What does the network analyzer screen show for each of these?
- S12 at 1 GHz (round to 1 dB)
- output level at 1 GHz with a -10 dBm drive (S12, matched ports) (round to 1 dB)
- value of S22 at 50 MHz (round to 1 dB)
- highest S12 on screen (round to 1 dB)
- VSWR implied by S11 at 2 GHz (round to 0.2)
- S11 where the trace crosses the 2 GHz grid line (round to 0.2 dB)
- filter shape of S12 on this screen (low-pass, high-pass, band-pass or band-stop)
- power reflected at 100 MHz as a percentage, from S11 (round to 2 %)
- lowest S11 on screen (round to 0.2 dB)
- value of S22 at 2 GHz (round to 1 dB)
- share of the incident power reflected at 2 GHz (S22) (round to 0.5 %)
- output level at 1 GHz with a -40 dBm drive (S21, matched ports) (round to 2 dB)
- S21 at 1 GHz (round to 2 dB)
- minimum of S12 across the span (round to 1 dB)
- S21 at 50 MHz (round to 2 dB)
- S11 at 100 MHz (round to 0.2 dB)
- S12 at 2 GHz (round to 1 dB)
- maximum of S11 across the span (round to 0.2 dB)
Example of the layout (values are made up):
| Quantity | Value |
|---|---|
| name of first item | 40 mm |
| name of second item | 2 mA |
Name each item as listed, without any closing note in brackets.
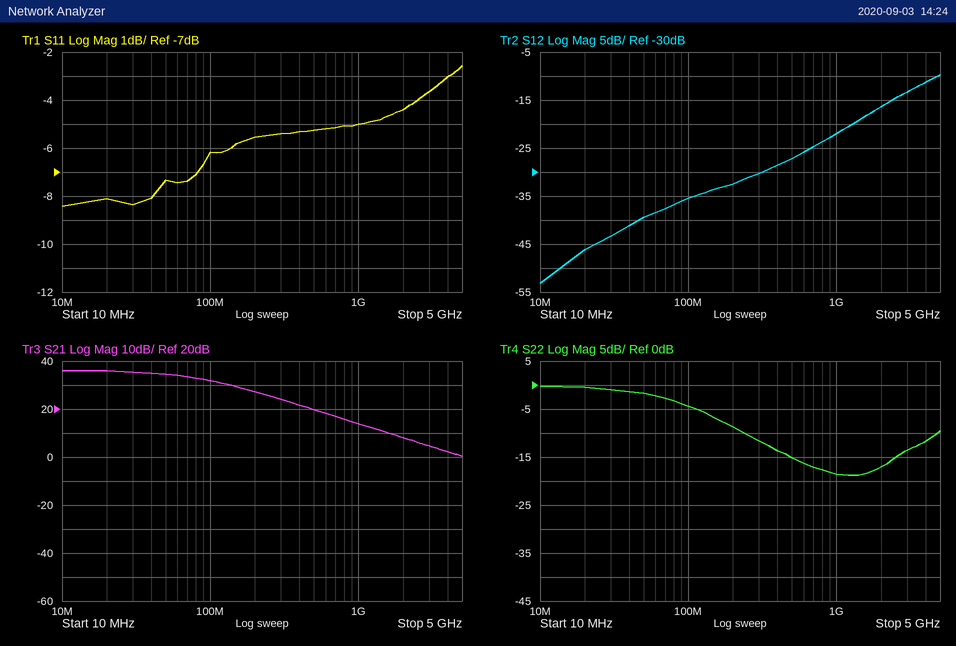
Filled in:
| Quantity | Value |
|---|---|
| S12 at 1 GHz | -22 dB |
| output level at 1 GHz with a -10 dBm drive (S12, matched ports) | -32 dBm |
| value of S22 at 50 MHz | -2 dB |
| highest S12 on screen | -10 dB |
| VSWR implied by S11 at 2 GHz | 4.0 |
| S11 where the trace crosses the 2 GHz grid line | -4.4 dB |
| filter shape of S12 on this screen | high-pass |
| power reflected at 100 MHz as a percentage, from S11 | 24 % |
| lowest S11 on screen | -8.4 dB |
| value of S22 at 2 GHz | -17 dB |
| share of the incident power reflected at 2 GHz (S22) | 2.0 % |
| output level at 1 GHz with a -40 dBm drive (S21, matched ports) | -26 dBm |
| S21 at 1 GHz | 14 dB |
| minimum of S12 across the span | -53 dB |
| S21 at 50 MHz | 34 dB |
| S11 at 100 MHz | -6.2 dB |
| S12 at 2 GHz | -16 dB |
| maximum of S11 across the span | -2.6 dB |
